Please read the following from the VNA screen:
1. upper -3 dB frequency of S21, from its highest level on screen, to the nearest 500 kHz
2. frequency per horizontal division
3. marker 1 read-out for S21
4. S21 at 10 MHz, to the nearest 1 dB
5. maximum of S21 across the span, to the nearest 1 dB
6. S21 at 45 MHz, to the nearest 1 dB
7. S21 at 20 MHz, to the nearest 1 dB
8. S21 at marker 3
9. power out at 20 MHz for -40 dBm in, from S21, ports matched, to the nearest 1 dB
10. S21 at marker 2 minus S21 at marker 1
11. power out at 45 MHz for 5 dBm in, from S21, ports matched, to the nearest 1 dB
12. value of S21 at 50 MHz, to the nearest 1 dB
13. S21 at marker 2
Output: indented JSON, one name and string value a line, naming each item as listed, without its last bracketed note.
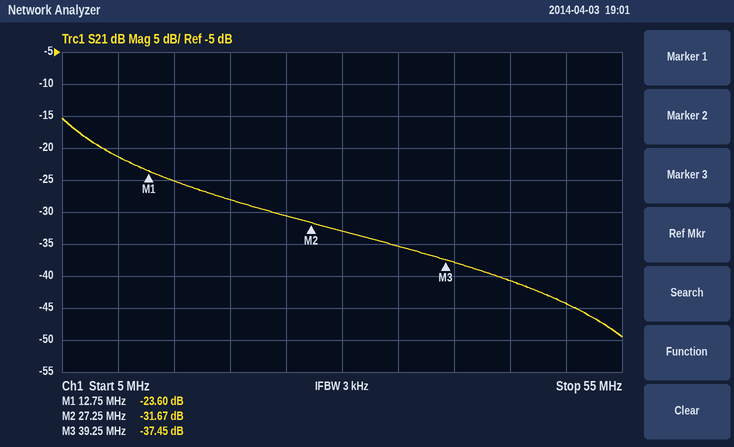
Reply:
{
  "upper -3 dB frequency of S21, from its highest level on screen, to the nearest 500 kHz": "7.0 MHz",
  "frequency per horizontal division": "5 MHz",
  "marker 1 read-out for S21": "-23.60 dB",
  "S21 at 10 MHz, to the nearest 1 dB": "-21 dB",
  "maximum of S21 across the span, to the nearest 1 dB": "-15 dB",
  "S21 at 45 MHz, to the nearest 1 dB": "-41 dB",
  "S21 at 20 MHz, to the nearest 1 dB": "-28 dB",
  "S21 at marker 3": "-37.45 dB",
  "power out at 20 MHz for -40 dBm in, from S21, ports matched, to the nearest 1 dB": "-68 dBm",
  "S21 at marker 2 minus S21 at marker 1": "-8.07 dB",
  "power out at 45 MHz for 5 dBm in, from S21, ports matched, to the nearest 1 dB": "-36 dBm",
  "value of S21 at 50 MHz, to the nearest 1 dB": "-44 dB",
  "S21 at marker 2": "-31.67 dB"
}
